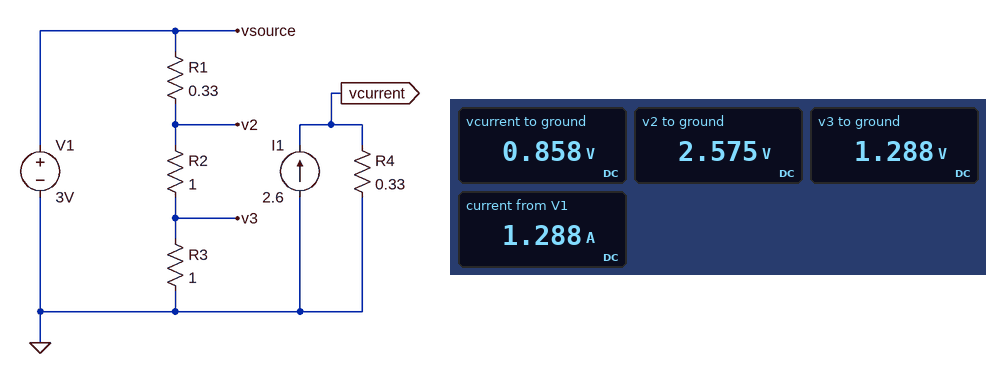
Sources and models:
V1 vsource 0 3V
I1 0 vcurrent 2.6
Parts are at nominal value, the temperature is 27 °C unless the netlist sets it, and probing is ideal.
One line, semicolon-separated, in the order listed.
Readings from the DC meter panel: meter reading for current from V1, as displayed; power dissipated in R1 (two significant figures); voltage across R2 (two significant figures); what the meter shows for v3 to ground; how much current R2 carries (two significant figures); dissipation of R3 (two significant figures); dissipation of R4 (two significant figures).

1.288 A; 550 mW; 1.3 V; 1.288 V; 1.3 A; 1.7 W; 2.2 W
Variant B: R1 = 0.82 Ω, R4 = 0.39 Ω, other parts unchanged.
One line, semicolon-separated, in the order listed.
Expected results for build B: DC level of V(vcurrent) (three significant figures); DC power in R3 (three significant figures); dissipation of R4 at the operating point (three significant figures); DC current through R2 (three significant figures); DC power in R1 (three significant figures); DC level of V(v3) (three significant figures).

1.01 V; 1.13 W; 2.64 W; 1.06 A; 928 mW; 1.06 V
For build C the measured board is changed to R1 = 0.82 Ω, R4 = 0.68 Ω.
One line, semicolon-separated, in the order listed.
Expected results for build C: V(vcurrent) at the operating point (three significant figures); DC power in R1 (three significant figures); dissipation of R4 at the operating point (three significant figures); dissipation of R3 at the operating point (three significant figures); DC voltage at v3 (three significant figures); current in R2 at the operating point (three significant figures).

1.77 V; 928 mW; 4.60 W; 1.13 W; 1.06 V; 1.06 A
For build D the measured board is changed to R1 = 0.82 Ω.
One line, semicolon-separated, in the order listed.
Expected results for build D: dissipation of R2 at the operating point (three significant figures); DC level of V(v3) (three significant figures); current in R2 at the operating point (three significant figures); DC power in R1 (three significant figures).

1.13 W; 1.06 V; 1.06 A; 928 mW
